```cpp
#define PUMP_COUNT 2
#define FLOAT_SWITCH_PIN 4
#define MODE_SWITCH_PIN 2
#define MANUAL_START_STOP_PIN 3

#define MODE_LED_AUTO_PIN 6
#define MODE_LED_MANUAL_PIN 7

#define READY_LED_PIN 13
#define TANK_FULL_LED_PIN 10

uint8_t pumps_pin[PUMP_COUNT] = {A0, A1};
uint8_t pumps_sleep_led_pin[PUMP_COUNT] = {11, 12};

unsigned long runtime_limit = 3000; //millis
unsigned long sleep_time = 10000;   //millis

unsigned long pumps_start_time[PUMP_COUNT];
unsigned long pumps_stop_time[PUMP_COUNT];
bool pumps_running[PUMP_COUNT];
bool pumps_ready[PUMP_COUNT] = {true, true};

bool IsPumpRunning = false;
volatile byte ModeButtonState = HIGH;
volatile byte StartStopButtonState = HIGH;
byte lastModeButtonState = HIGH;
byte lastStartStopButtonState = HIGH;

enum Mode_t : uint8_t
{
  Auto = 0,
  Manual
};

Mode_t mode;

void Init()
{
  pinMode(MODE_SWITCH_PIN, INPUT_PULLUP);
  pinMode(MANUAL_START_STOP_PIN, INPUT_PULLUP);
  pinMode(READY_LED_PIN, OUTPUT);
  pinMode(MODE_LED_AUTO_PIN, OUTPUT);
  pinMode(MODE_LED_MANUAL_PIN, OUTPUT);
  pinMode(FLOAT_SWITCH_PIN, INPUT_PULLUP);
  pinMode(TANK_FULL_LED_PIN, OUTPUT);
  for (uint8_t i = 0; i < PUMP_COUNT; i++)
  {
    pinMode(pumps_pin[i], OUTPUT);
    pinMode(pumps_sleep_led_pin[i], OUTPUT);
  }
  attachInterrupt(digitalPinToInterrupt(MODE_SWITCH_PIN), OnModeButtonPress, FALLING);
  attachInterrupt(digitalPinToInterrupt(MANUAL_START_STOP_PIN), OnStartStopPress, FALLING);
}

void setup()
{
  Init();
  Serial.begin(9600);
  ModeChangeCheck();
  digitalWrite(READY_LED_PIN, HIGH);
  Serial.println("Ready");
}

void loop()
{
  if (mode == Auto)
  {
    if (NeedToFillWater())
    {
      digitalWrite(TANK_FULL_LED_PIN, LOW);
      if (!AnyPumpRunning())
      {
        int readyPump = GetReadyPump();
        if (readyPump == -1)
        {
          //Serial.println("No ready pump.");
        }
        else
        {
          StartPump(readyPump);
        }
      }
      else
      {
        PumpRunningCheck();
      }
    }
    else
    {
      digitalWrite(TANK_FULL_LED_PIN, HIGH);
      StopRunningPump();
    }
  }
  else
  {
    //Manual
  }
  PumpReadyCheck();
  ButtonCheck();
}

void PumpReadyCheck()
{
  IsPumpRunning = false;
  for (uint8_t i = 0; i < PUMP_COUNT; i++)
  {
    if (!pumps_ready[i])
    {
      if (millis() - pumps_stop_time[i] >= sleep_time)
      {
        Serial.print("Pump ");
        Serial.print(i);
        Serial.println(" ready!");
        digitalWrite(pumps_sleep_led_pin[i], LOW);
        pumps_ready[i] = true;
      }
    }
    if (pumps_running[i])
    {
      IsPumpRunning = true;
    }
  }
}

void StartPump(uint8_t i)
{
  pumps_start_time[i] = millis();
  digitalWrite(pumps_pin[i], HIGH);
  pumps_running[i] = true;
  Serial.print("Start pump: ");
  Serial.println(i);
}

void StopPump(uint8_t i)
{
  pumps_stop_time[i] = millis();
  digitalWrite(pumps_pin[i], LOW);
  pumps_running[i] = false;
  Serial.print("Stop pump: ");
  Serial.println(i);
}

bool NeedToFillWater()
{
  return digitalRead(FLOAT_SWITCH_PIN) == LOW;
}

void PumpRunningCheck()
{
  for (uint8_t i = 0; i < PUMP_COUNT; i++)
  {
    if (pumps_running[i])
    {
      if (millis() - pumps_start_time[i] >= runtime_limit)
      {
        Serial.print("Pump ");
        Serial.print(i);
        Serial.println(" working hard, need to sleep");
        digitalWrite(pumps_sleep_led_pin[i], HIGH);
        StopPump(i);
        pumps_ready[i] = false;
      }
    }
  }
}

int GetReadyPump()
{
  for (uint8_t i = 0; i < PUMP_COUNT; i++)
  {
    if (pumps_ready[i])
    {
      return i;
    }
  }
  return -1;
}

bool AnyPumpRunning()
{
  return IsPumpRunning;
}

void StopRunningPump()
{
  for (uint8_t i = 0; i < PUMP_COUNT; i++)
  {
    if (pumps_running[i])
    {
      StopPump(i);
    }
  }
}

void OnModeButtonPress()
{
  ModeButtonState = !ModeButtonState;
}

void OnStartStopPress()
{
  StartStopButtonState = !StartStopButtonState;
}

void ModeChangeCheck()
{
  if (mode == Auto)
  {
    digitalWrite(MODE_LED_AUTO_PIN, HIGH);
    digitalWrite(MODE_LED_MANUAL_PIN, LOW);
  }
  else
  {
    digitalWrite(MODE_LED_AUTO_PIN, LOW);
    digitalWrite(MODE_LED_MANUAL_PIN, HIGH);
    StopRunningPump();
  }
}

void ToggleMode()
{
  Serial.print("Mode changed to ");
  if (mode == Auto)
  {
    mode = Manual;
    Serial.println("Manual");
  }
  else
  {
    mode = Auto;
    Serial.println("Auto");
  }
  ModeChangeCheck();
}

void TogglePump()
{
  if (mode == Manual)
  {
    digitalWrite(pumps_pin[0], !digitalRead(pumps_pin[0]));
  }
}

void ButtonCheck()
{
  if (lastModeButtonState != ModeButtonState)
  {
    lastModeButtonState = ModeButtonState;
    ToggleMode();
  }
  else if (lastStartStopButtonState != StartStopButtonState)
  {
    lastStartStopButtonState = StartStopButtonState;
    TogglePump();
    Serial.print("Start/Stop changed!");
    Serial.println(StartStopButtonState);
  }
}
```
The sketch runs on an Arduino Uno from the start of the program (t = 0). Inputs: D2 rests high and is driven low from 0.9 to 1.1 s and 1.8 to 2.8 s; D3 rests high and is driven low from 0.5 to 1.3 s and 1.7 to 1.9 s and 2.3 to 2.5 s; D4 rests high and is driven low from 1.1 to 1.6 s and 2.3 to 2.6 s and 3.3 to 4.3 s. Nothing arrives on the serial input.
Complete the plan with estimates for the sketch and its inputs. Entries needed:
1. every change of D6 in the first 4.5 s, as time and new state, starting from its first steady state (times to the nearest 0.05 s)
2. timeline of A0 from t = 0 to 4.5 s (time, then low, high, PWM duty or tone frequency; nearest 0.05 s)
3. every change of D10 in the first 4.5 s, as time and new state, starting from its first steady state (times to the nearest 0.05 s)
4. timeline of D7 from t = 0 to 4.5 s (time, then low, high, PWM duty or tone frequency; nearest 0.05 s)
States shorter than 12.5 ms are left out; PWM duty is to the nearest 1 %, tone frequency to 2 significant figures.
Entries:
0 s high; 0.9 s low; 1.8 s high
0 s low; 1.7 s high; 2.6 s low; 3.3 s high; 4.3 s low
0 s high; 2.3 s low; 2.6 s high; 3.3 s low; 4.3 s high
0 s low; 0.9 s high; 1.8 s low
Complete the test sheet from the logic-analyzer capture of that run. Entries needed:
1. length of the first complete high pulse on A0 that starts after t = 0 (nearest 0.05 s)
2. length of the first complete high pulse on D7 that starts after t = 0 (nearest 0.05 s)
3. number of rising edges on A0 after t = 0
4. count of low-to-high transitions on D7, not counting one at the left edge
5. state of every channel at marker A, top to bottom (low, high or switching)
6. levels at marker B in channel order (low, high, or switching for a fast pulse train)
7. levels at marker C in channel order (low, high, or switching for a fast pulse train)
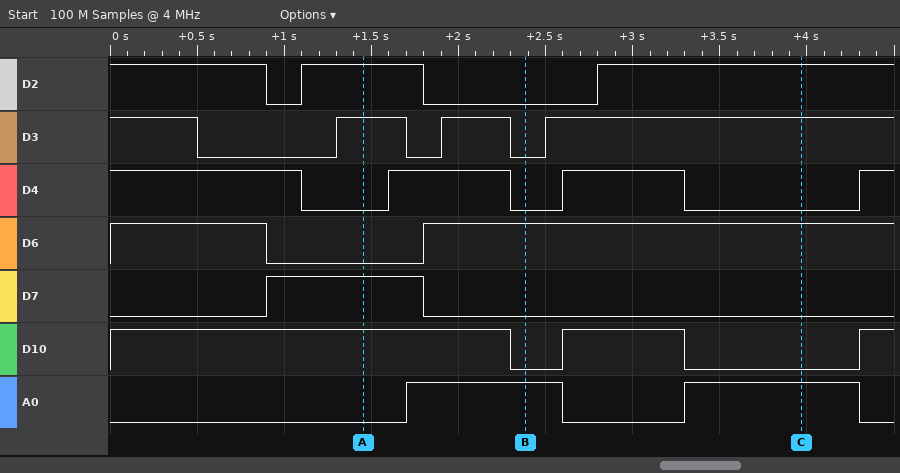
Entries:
0.90 s
0.90 s
2
1
D2 high, D3 high, D4 low, D6 low, D7 high, D10 high, A0 low
D2 low, D3 low, D4 low, D6 high, D7 low, D10 low, A0 high
D2 high, D3 high, D4 low, D6 high, D7 low, D10 low, A0 high
